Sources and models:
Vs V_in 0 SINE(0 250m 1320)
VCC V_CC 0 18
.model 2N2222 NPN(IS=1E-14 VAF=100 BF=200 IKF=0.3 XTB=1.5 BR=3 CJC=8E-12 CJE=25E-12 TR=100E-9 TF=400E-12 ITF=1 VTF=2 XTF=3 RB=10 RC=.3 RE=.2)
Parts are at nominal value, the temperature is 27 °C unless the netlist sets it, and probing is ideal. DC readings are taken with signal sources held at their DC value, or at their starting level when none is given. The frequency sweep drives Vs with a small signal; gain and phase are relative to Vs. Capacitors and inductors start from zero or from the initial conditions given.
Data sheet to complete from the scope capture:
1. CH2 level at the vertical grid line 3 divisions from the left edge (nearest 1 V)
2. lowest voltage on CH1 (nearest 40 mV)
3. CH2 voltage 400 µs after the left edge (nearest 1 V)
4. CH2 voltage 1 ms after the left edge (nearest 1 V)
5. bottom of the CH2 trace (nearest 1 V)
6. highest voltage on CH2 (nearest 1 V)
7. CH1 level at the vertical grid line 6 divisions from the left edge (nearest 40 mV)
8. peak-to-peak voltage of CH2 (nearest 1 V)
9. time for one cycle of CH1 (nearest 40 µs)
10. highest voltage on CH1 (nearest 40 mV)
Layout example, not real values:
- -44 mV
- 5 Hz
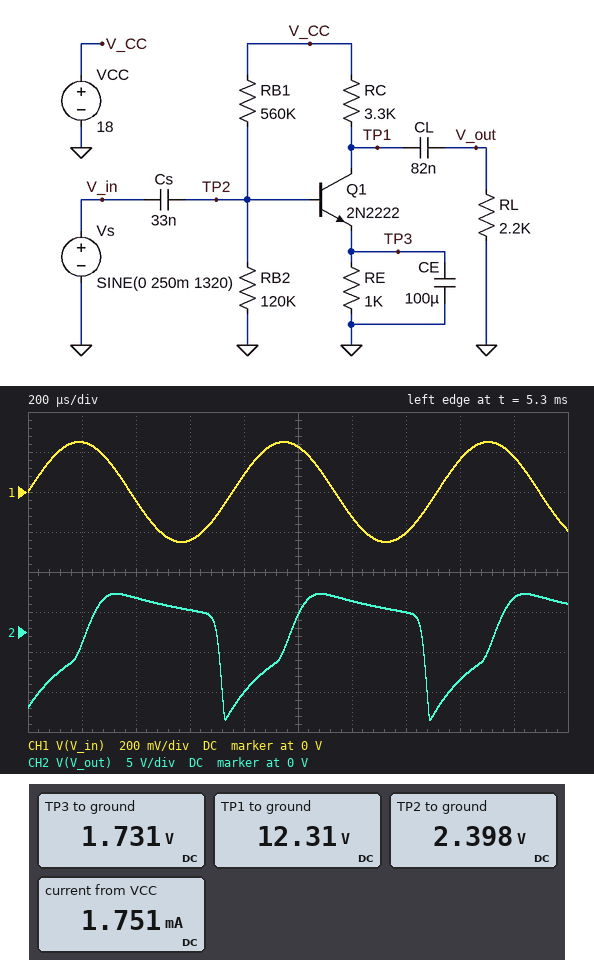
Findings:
- 3 V
- -240 mV
- 4 V
- 2 V
- -11 V
- 5 V
- -120 mV
- 16 V
- 760 µs
- 240 mV
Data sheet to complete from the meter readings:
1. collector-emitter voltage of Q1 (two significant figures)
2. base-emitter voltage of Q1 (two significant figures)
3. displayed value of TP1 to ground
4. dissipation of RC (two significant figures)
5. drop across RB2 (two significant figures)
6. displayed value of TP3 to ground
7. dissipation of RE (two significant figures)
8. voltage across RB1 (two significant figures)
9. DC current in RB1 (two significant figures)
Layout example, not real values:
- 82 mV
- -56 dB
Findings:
- 11 V
- 670 mV
- 12.31 V
- 9.8 mW
- 2.4 V
- 1.731 V
- 3.0 mW
- 16 V
- 28 µA
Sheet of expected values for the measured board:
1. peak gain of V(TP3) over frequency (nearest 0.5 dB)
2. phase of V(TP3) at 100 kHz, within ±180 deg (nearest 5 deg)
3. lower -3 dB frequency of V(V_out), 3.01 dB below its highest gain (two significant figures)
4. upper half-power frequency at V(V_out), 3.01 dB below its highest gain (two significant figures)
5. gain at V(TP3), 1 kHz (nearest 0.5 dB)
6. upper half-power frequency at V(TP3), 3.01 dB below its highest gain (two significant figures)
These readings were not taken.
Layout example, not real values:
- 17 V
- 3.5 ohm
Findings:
- -24.0 dB
- -90 deg
- 1.7 kHz
- 22 MHz
- -25.5 dB
- 1.7 kHz
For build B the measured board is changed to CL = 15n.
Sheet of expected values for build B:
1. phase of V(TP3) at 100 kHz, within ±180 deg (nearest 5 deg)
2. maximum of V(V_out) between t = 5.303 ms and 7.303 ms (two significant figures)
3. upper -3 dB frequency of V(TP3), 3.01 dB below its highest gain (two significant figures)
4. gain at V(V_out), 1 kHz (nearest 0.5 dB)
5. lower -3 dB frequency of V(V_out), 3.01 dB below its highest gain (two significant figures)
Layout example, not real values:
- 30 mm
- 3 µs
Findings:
- -90 deg
- 3.4 V
- 1.6 kHz
- 26.0 dB
- 2.8 kHz
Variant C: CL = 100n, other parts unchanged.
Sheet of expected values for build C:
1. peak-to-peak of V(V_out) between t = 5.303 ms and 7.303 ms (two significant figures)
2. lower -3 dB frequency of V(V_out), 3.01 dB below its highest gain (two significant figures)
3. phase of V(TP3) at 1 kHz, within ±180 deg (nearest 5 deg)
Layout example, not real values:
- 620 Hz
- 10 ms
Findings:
- 15 V
- 1.6 kHz
- -30 deg
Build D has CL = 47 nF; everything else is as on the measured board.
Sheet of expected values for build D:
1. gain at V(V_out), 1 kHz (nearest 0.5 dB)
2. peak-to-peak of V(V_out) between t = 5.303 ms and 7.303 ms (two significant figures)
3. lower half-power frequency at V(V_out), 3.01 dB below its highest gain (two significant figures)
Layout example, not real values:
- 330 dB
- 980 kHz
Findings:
- 31.5 dB
- 17 V
- 1.8 kHz
